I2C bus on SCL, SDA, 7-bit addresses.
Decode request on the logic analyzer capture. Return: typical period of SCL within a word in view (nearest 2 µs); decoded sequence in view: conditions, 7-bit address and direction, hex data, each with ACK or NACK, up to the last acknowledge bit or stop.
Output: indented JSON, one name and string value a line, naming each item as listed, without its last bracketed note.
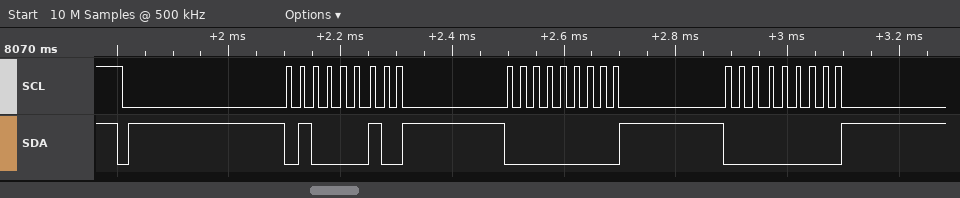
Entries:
{
  "typical period of SCL within a word in view": "24 µs",
  "decoded sequence in view: conditions, 7-bit address and direction, hex data, each with ACK or NACK, up to the last acknowledge bit or stop": "start, address 21 write ACK, 00 ACK, 00 ACK"
}
